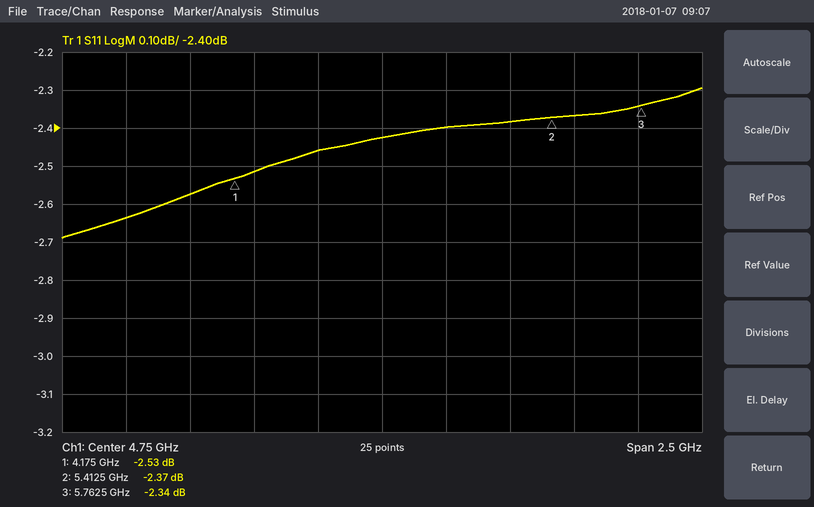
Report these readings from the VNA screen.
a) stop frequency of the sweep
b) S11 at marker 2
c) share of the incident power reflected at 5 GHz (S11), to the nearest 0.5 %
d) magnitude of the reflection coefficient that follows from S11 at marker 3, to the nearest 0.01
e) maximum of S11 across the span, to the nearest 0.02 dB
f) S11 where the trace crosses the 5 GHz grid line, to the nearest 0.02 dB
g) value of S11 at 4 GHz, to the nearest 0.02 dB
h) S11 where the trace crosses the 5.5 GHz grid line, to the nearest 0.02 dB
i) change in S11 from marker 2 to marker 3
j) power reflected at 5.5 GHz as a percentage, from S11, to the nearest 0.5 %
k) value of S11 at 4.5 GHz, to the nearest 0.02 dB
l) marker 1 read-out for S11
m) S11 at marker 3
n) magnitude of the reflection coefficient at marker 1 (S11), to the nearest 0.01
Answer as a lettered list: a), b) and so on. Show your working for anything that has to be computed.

a) 6 GHz
b) -2.37 dB
c) 10^(-2.4/10) ≈ 57.5 %
d) 10^(-2.34/20) ≈ 0.76
e) -2.30 dB
f) -2.40 dB
g) -2.58 dB
h) -2.36 dB
i) -2.34 − (-2.37) = 0.03 dB
j) 10^(-2.36/10) ≈ 58.1 %, so 58.0 % to the nearest 0.5 %
k) -2.46 dB
l) -2.53 dB
m) -2.34 dB
n) 10^(-2.53/20) ≈ 0.75
